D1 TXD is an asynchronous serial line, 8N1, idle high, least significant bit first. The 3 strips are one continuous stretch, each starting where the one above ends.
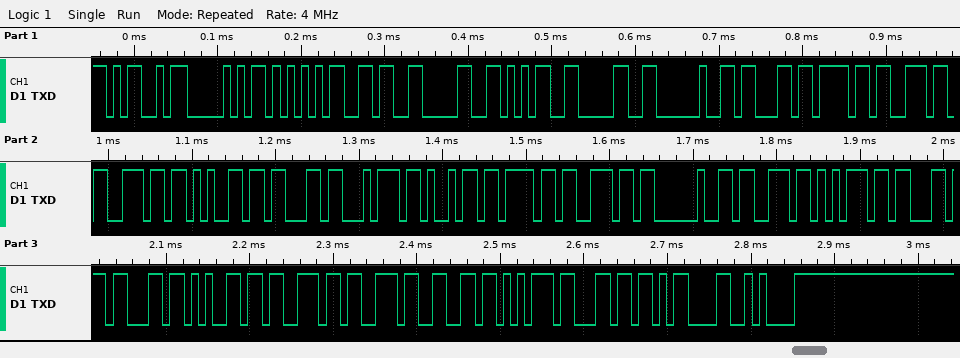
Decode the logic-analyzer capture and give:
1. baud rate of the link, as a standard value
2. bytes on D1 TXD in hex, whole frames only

115200 baud
0x4D 0x50 0x55 0x36 0x30 0x35 0x30 0x20 0x63 0x6F 0x6E 0x6E 0x65 0x63 0x74 0x69 0x6F 0x6E 0x20 0x73 0x75 0x63 0x63 0x65 0x73 0x73 0x66 0x75 0x6C 0x0D 0x0A
